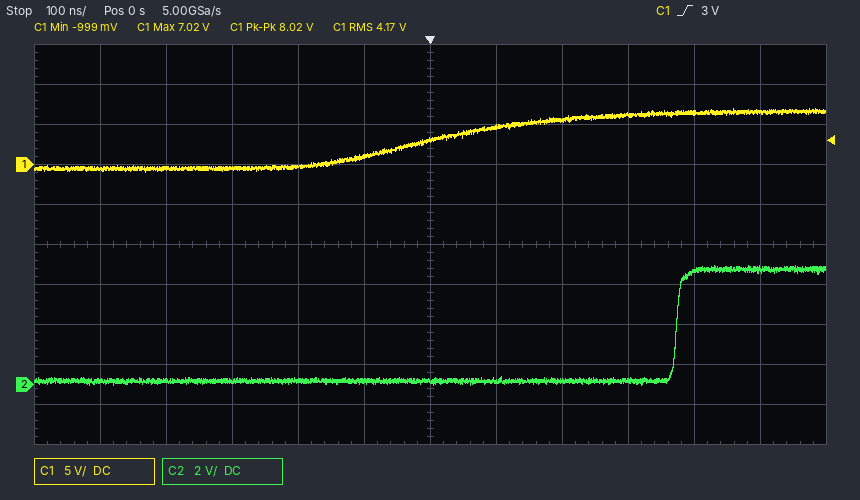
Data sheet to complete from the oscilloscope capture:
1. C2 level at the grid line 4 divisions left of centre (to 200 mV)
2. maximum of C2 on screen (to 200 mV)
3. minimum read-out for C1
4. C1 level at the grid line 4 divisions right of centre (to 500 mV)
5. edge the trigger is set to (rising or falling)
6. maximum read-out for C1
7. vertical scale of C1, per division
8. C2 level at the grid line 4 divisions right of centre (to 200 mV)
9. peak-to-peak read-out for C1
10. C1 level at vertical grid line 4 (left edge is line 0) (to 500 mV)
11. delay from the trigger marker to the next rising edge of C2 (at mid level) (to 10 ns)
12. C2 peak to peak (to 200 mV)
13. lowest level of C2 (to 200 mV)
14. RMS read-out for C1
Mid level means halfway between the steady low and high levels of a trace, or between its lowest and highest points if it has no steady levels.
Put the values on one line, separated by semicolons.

200 mV; 6.0 V; -999 mV; 6.5 V; rising; 7.02 V; 5 V; 5.6 V; 8.02 V; -500 mV; 370 ns; 6.0 V; 0.0 V; 4.17 V
